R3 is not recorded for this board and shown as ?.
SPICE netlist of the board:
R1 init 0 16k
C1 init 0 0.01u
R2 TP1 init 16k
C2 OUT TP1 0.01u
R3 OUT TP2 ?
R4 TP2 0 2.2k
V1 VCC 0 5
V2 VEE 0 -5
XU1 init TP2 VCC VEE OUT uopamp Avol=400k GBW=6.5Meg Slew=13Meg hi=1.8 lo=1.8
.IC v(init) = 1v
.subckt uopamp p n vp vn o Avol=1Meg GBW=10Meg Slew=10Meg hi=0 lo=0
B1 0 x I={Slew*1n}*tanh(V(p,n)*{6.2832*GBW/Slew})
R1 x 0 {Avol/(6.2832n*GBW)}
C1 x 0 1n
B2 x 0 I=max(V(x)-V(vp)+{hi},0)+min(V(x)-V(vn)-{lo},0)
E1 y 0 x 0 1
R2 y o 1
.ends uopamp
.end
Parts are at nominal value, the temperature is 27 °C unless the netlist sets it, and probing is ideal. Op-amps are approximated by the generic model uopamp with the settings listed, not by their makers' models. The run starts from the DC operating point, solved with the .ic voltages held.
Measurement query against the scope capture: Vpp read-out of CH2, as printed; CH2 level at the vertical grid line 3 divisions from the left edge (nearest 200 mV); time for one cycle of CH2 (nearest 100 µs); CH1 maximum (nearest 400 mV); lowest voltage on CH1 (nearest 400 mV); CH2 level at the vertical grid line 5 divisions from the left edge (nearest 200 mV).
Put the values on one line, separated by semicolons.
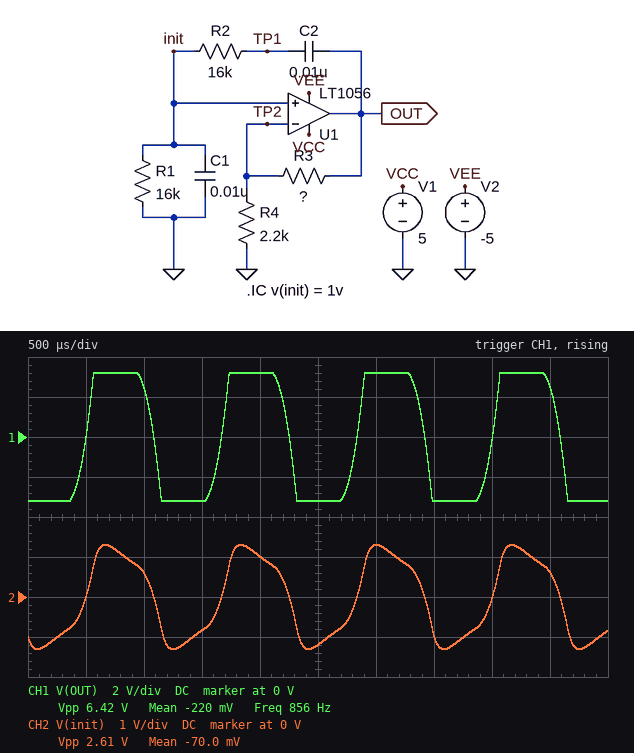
2.61 V; -800 mV; 1.2 ms; 3.2 V; -3.2 V; -1.2 V
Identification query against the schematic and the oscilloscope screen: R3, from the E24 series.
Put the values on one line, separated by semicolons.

6.8 kΩ
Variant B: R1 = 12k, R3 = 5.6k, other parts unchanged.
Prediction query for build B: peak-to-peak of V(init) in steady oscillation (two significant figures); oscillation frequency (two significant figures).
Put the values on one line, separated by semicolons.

2.1 V; 1.1 kHz
